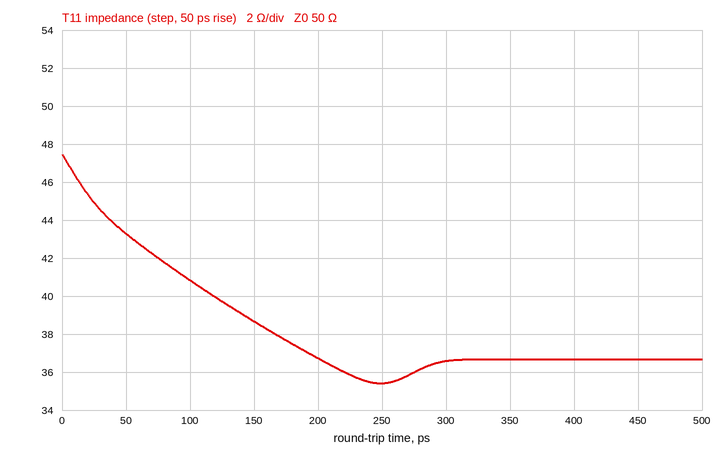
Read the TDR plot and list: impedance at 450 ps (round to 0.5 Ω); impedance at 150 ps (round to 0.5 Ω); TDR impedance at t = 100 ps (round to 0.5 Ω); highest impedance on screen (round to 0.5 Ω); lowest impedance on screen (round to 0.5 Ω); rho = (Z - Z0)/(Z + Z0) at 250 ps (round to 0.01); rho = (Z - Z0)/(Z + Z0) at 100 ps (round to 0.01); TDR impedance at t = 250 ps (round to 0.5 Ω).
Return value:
36.5 Ω
38.5 Ω
41.0 Ω
47.5 Ω
35.5 Ω
-0.17
-0.10
35.5 Ω
